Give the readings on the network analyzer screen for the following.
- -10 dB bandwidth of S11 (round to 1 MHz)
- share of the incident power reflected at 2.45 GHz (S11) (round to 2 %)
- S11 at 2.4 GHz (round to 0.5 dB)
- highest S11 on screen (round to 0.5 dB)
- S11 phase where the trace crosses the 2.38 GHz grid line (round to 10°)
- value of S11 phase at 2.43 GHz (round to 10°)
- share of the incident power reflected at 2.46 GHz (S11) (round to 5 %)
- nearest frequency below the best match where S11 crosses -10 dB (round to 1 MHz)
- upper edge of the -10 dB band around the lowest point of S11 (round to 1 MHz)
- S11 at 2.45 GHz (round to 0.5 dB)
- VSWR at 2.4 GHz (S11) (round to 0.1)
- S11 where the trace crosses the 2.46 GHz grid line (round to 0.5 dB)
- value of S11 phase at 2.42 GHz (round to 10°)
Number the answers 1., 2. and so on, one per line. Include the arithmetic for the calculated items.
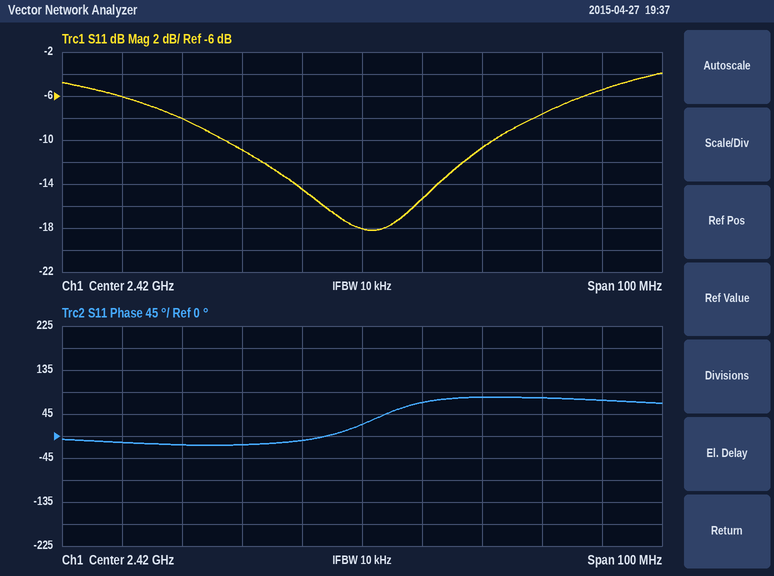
1. 2.442 GHz − 2.397 GHz = 45 MHz
2. 10^(-7.5/10) ≈ 18 %
3. -11.0 dB
4. -4.0 dB
5. -10°
6. 70°
7. 10^(-5.5/10) ≈ 28.2 %, so 30 % to the nearest 5 %
8. 2.397 GHz
9. 2.442 GHz
10. -7.5 dB
11. |Γ| = 10^(-11/20) = 0.2818; VSWR = (1 + 0.2818)/(1 − 0.2818) ≈ 1.8
12. -5.5 dB
13. 20°
